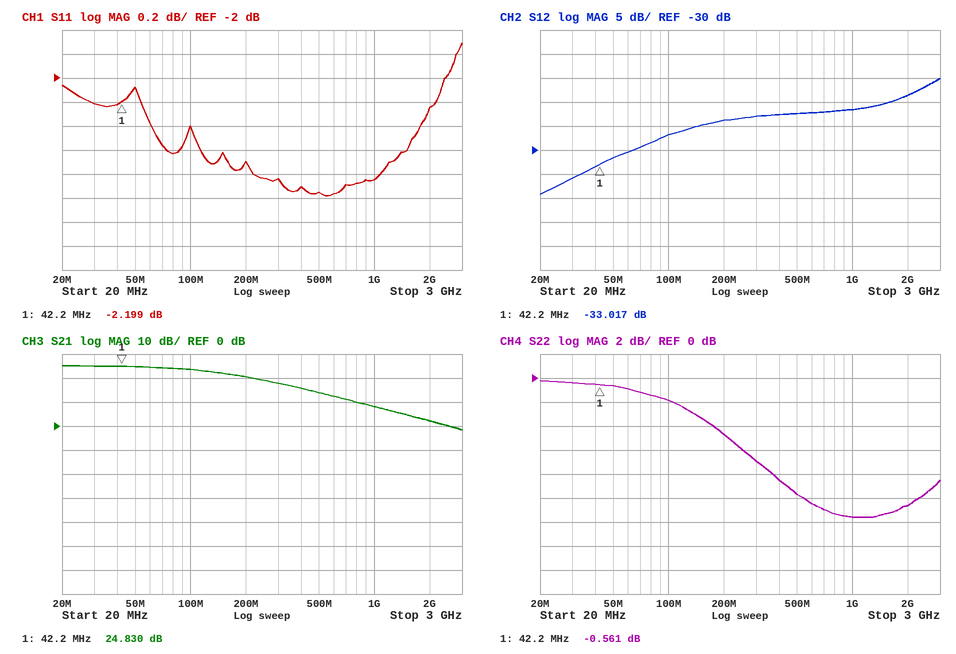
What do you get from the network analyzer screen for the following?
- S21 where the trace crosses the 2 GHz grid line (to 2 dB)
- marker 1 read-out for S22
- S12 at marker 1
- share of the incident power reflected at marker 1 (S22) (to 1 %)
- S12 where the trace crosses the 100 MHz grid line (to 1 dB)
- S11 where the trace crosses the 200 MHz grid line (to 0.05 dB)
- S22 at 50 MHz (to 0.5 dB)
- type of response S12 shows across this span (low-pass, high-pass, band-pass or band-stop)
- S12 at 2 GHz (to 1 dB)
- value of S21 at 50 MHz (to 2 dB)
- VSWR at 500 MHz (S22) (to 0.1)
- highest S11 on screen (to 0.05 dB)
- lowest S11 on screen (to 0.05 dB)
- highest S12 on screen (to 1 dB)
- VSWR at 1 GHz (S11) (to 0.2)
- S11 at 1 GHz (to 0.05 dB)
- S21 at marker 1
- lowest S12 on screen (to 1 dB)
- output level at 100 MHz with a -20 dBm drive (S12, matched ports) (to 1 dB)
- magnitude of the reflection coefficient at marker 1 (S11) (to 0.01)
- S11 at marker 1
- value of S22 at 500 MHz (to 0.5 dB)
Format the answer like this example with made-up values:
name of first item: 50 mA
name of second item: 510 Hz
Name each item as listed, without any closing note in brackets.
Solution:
S21 where the trace crosses the 2 GHz grid line: 2 dB
marker 1 read-out for S22: -0.561 dB
S12 at marker 1: -33.017 dB
share of the incident power reflected at marker 1 (S22): 88 %
S12 where the trace crosses the 100 MHz grid line: -27 dB
S11 where the trace crosses the 200 MHz grid line: -2.70 dB
S22 at 50 MHz: -0.5 dB
type of response S12 shows across this span: high-pass
S12 at 2 GHz: -19 dB
value of S21 at 50 MHz: 24 dB
VSWR at 500 MHz (S22): 2.0
highest S11 on screen: -1.70 dB
lowest S11 on screen: -3.00 dB
highest S12 on screen: -15 dB
VSWR at 1 GHz (S11): 6.2
S11 at 1 GHz: -2.85 dB
S21 at marker 1: 24.830 dB
lowest S12 on screen: -39 dB
output level at 100 MHz with a -20 dBm drive (S12, matched ports): -47 dBm
magnitude of the reflection coefficient at marker 1 (S11): 0.78
S11 at marker 1: -2.199 dB
value of S22 at 500 MHz: -9.5 dB
